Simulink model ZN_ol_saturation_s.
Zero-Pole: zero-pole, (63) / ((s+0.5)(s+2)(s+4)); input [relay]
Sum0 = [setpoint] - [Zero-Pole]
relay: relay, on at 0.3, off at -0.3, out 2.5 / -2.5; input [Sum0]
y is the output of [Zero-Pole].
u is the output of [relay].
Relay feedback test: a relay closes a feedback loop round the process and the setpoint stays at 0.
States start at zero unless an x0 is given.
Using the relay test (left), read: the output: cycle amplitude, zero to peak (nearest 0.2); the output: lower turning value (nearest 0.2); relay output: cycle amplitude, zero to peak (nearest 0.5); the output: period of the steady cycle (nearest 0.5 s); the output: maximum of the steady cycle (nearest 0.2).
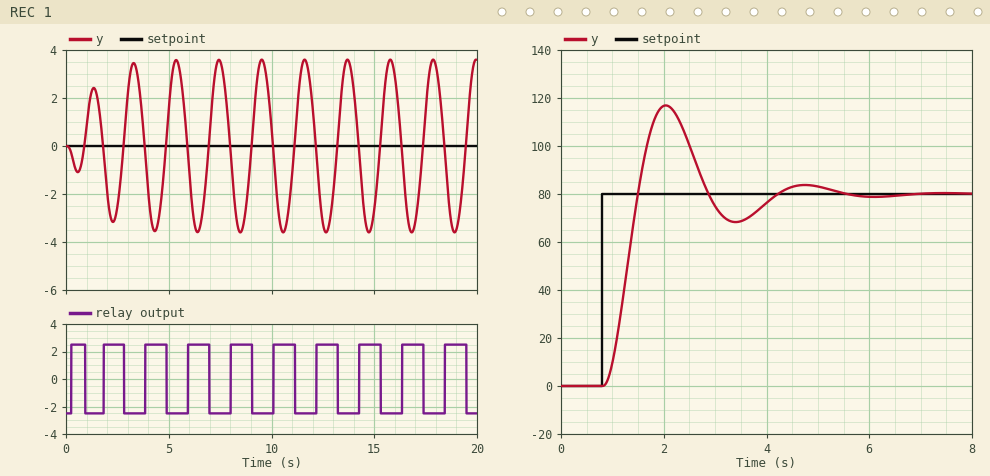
3.6
-3.6
2.5
2.0 s
3.6
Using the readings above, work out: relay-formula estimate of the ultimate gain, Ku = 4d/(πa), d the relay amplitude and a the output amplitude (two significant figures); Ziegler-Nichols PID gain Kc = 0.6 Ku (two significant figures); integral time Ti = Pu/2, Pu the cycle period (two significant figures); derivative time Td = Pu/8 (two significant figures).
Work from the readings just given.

0.88
0.53
1.0 s
0.25 s
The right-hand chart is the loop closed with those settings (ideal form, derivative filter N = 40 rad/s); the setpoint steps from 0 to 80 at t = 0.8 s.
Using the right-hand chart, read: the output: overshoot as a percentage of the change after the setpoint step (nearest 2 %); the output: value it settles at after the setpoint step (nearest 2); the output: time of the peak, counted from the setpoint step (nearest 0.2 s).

46 %
80
1.2 s
